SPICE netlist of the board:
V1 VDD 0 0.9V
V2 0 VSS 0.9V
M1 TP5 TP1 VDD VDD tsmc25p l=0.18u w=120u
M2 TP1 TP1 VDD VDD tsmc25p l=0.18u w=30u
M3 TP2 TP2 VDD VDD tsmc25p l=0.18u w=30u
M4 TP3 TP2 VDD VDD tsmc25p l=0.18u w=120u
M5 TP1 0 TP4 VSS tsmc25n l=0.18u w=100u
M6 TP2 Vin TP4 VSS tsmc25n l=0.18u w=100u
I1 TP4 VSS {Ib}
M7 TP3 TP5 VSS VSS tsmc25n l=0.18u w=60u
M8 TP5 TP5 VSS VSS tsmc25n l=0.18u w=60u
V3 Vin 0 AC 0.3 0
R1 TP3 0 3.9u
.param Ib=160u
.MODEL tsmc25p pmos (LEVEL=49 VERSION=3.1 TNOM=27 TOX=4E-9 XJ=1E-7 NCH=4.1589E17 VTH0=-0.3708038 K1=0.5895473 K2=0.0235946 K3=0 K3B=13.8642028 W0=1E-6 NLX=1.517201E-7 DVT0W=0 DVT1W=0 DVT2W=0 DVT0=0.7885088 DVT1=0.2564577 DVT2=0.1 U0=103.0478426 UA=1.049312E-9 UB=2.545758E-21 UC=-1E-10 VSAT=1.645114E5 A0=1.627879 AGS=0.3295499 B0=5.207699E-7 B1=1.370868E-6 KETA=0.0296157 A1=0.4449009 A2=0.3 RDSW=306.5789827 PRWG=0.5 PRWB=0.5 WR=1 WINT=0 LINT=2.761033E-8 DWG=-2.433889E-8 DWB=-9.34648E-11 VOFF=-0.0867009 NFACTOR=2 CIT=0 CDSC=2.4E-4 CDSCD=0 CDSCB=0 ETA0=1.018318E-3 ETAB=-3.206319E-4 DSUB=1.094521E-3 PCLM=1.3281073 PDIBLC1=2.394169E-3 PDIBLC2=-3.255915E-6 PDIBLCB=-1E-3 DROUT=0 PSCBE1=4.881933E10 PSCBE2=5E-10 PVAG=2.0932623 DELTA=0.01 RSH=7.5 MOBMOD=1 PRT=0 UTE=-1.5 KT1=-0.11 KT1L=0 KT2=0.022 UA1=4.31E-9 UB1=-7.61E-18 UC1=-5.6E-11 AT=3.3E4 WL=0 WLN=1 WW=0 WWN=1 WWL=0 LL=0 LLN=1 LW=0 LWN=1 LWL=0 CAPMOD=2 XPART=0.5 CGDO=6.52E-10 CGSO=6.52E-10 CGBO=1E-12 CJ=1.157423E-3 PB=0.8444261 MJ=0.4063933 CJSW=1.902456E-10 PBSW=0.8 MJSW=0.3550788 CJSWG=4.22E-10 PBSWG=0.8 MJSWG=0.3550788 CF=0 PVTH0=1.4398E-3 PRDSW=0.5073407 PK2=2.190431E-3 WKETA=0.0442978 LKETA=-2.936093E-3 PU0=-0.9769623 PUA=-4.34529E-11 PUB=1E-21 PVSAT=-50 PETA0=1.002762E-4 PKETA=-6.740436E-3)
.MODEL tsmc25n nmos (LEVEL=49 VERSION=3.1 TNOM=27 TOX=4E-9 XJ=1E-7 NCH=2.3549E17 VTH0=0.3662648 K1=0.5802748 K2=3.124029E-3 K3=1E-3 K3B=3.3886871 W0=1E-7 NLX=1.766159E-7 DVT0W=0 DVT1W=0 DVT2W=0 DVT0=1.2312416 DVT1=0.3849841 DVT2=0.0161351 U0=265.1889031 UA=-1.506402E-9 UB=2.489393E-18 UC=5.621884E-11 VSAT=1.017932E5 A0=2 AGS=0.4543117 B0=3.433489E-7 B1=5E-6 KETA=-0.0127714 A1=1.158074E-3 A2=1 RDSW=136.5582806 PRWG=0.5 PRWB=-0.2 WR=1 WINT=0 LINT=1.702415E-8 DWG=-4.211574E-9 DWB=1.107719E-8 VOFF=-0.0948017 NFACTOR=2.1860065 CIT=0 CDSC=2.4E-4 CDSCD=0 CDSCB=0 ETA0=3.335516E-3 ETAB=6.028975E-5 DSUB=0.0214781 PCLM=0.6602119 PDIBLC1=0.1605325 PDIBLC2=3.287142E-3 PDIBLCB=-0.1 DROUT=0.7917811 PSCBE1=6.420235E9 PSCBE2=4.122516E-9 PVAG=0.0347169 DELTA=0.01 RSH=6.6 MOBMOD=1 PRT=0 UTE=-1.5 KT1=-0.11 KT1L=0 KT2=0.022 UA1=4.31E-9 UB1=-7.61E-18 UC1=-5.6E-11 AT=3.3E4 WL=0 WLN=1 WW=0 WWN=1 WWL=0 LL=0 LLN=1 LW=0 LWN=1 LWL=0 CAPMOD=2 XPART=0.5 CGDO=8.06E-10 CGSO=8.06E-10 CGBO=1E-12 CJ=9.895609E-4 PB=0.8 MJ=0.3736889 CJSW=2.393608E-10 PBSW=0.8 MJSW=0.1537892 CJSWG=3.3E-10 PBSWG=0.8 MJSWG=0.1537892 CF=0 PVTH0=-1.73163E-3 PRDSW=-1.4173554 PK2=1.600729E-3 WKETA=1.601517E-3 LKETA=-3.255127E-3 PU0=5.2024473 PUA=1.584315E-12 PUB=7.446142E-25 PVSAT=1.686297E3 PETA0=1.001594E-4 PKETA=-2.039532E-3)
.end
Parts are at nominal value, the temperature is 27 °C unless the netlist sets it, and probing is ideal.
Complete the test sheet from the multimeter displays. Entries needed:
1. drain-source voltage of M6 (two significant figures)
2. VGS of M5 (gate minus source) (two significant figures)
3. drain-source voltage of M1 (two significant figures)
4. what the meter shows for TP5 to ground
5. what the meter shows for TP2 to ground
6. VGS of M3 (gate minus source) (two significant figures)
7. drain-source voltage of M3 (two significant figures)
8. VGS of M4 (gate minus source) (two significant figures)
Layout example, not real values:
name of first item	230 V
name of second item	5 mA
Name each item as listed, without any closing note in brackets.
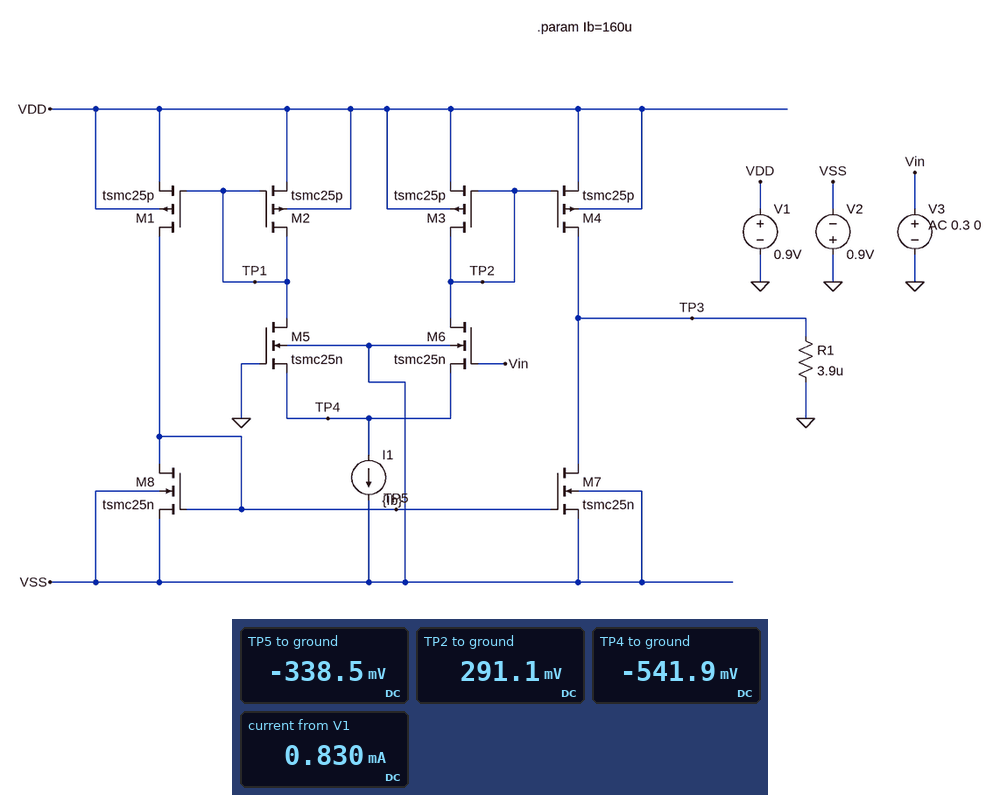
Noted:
drain-source voltage of M6	830 mV
VGS of M5 (gate minus source)	540 mV
drain-source voltage of M1	-1.2 V
what the meter shows for TP5 to ground	-338.5 mV
what the meter shows for TP2 to ground	291.1 mV
VGS of M3 (gate minus source)	-610 mV
drain-source voltage of M3	-610 mV
VGS of M4 (gate minus source)	-610 mV
